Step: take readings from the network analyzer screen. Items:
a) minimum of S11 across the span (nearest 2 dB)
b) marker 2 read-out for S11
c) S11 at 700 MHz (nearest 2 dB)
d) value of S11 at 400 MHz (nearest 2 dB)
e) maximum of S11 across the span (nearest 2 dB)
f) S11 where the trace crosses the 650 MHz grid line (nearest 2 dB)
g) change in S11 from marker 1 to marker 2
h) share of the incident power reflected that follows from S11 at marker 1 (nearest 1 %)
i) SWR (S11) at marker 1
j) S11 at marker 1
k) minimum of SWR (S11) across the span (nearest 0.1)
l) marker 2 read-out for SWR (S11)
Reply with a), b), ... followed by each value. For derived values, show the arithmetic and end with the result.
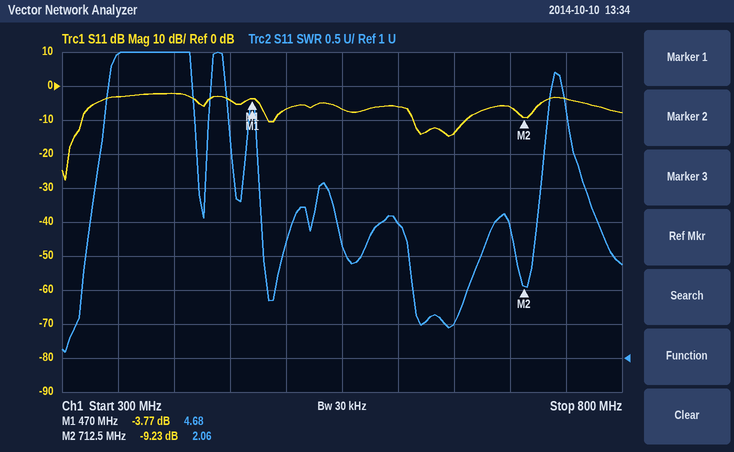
a) -28 dB
b) -9.23 dB
c) -6 dB
d) -2 dB
e) -2 dB
f) -14 dB
g) -9.23 − (-3.77) = -5.46 dB
h) 10^(-3.77/10) ≈ 42 %
i) 4.68
j) -3.77 dB
k) 1.1
l) 2.06
